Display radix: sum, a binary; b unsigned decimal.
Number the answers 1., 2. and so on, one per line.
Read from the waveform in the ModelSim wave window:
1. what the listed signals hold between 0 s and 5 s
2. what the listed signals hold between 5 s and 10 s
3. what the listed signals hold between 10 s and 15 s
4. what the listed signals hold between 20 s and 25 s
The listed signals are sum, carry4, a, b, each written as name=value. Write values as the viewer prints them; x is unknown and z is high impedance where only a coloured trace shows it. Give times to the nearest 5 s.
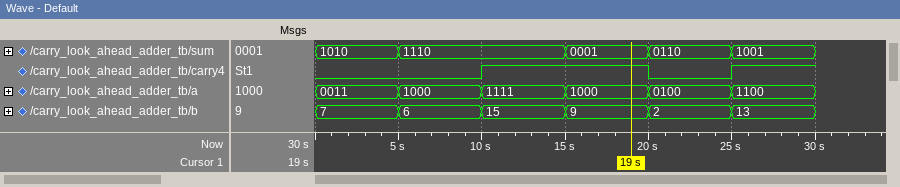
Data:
1. sum=1010, carry4=0, a=0011, b=7
2. sum=1110, carry4=0, a=1000, b=6
3. sum=1110, carry4=1, a=1111, b=15
4. sum=0110, carry4=0, a=0100, b=2
